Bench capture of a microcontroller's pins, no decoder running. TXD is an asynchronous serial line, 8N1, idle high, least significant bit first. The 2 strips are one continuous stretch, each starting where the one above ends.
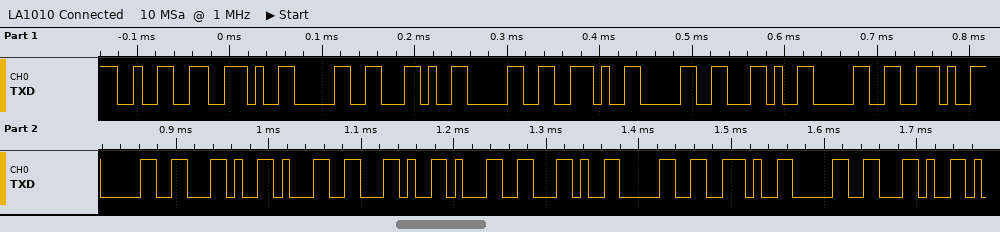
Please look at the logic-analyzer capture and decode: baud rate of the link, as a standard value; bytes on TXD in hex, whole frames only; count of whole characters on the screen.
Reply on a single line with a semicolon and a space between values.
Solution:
115200 baud; 32 2E 30 2C 30 2E 30 2C 30 2E 30 2C 31 2C 31 2C 30 2E 30 2C; 20
